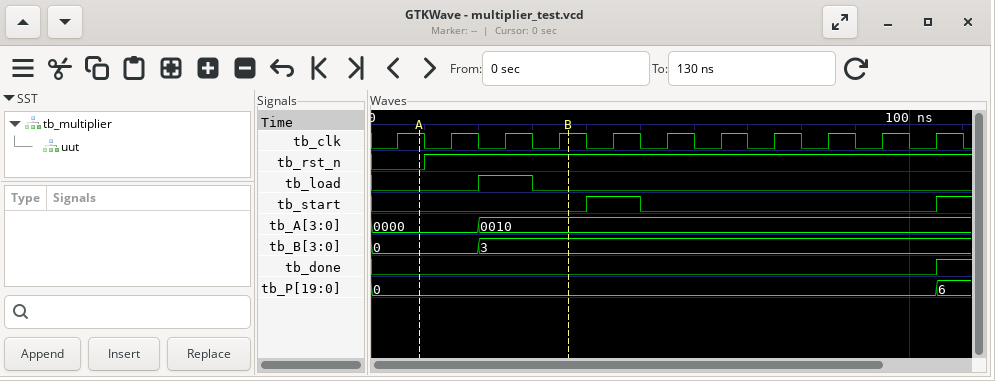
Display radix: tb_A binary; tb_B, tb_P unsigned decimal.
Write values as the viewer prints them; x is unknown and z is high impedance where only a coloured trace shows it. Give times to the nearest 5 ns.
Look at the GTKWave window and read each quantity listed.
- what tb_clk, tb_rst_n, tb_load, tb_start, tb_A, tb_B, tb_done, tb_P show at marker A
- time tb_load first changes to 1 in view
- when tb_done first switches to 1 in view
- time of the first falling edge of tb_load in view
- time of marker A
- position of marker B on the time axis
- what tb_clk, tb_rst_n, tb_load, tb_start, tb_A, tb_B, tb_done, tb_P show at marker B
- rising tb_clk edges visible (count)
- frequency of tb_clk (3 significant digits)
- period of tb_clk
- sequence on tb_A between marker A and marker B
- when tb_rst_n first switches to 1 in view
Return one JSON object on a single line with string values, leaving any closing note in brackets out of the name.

{"what tb_clk, tb_rst_n, tb_load, tb_start, tb_A, tb_B, tb_done, tb_P show at marker A": "tb_clk=1, tb_rst_n=0, tb_load=0, tb_start=0, tb_A=0000, tb_B=0, tb_done=0, tb_P=0", "time tb_load first changes to 1 in view": "20 ns", "when tb_done first switches to 1 in view": "105 ns", "time of the first falling edge of tb_load in view": "30 ns", "time of marker A": "10 ns", "position of marker B on the time axis": "35 ns", "what tb_clk, tb_rst_n, tb_load, tb_start, tb_A, tb_B, tb_done, tb_P show at marker B": "tb_clk=1, tb_rst_n=1, tb_load=0, tb_start=0, tb_A=0010, tb_B=3, tb_done=0, tb_P=0", "rising tb_clk edges visible": "11", "frequency of tb_clk": "100 MHz", "period of tb_clk": "10 ns", "sequence on tb_A between marker A and marker B": "0000, 0010", "when tb_rst_n first switches to 1 in view": "10 ns"}
